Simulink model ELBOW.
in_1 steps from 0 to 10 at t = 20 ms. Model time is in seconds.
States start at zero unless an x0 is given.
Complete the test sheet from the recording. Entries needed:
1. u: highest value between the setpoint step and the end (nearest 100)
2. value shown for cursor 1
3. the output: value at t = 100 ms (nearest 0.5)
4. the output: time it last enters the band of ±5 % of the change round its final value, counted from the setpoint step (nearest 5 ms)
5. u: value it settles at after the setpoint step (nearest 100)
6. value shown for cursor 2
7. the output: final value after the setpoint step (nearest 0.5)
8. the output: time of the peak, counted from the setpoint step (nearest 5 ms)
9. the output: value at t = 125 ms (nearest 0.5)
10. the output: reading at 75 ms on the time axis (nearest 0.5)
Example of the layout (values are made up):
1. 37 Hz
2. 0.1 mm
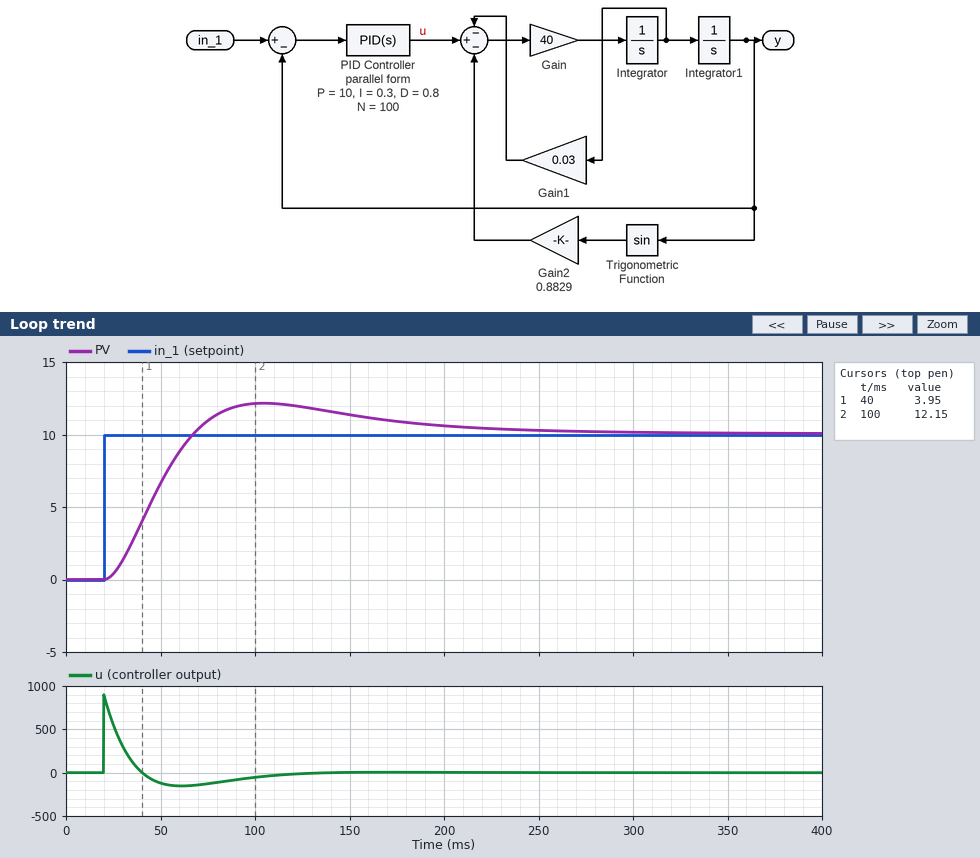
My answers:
1. 900
2. 3.95
3. 12.0
4. 185 ms
5. 0
6. 12.15
7. 10.0
8. 85 ms
9. 12.0
10. 11.0
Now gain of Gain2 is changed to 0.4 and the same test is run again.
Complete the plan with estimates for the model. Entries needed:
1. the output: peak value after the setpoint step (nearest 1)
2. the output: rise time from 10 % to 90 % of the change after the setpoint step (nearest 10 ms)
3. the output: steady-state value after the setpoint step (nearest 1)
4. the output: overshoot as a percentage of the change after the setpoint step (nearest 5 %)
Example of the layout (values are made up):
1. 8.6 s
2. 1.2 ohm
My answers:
1. 12
2. 30 ms
3. 10
4. 20 %
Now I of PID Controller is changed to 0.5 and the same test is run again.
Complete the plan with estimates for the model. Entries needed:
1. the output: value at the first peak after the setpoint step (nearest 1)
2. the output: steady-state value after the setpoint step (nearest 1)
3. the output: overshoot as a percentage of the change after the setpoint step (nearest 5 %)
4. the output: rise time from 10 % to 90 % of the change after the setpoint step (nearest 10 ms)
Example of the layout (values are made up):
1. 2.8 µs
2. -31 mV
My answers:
1. 12
2. 10
3. 20 %
4. 30 ms
